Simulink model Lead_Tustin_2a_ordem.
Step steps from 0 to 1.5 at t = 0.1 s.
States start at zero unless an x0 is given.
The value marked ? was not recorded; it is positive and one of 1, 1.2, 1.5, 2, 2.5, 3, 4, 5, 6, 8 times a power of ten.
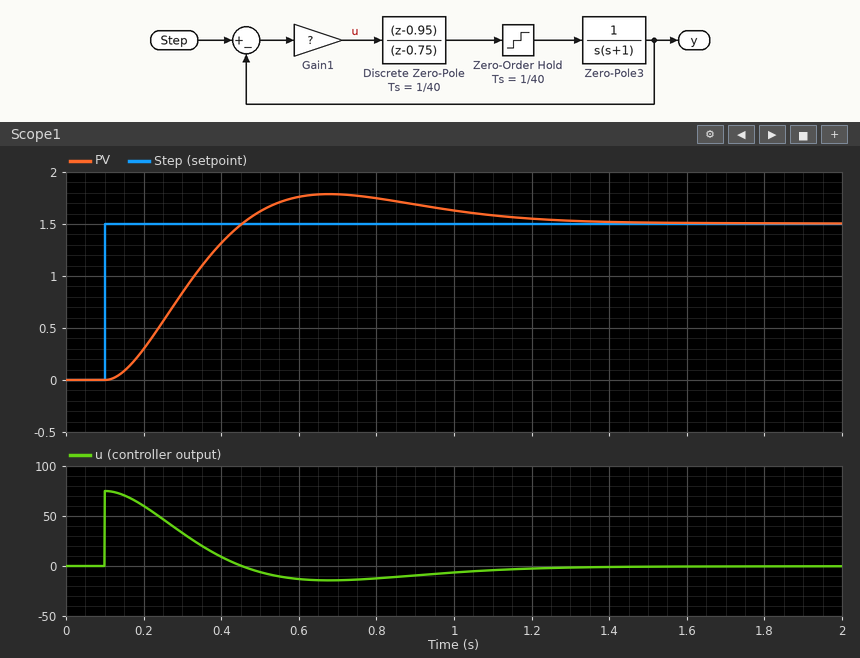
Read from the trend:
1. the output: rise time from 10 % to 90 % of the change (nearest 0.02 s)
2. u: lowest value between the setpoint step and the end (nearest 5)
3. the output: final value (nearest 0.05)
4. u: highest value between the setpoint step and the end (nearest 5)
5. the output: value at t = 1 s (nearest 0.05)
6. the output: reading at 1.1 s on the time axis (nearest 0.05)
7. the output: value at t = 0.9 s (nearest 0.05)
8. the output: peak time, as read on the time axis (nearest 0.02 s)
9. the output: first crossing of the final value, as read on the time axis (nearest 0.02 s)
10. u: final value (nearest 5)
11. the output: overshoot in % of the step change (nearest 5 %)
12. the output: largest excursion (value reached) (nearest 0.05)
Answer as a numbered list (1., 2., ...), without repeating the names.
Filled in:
1. 0.24 s
2. -15
3. 1.50
4. 75
5. 1.65
6. 1.60
7. 1.70
8. 0.68 s
9. 0.46 s
10. 0
11. 20 %
12. 1.80
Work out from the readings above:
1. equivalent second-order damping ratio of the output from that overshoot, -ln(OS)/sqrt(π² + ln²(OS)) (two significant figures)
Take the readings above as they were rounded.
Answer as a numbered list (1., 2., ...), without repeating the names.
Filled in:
1. 0.46
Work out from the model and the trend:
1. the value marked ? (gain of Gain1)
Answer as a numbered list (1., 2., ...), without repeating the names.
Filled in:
1. 50
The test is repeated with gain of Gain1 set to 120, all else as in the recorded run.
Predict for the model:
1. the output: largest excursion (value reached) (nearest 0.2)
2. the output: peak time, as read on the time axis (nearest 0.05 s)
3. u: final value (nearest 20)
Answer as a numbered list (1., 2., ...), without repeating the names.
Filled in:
1. 2.0
2. 0.40 s
3. 0
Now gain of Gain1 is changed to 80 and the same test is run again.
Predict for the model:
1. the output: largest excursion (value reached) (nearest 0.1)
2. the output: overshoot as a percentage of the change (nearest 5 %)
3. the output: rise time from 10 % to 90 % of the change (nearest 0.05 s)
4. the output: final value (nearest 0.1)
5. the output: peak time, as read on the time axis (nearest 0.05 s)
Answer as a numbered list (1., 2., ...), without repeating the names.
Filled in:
1. 1.9
2. 25 %
3. 0.15 s
4. 1.5
5. 0.50 s
